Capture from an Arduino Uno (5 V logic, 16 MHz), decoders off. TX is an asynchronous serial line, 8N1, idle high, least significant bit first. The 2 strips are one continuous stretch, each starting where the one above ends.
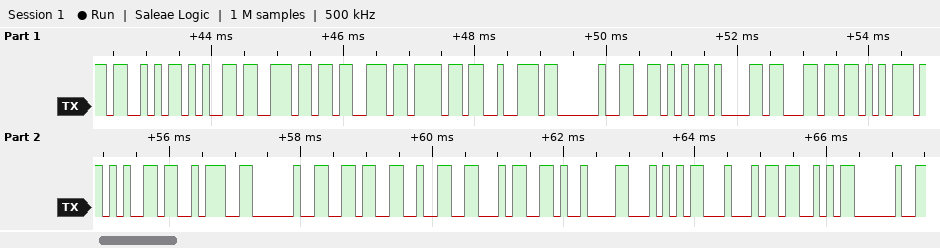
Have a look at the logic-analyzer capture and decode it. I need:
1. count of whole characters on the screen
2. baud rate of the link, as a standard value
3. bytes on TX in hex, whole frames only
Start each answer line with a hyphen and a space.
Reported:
- 22
- 9600 baud
- 0x53 0x65 0x6E 0x73 0x6F 0x72 0x20 0x56 0x61 0x6C 0x75 0x65 0x3A 0x20 0x36 0x32 0x34 0x09 0x54 0x44 0x53 0x20
